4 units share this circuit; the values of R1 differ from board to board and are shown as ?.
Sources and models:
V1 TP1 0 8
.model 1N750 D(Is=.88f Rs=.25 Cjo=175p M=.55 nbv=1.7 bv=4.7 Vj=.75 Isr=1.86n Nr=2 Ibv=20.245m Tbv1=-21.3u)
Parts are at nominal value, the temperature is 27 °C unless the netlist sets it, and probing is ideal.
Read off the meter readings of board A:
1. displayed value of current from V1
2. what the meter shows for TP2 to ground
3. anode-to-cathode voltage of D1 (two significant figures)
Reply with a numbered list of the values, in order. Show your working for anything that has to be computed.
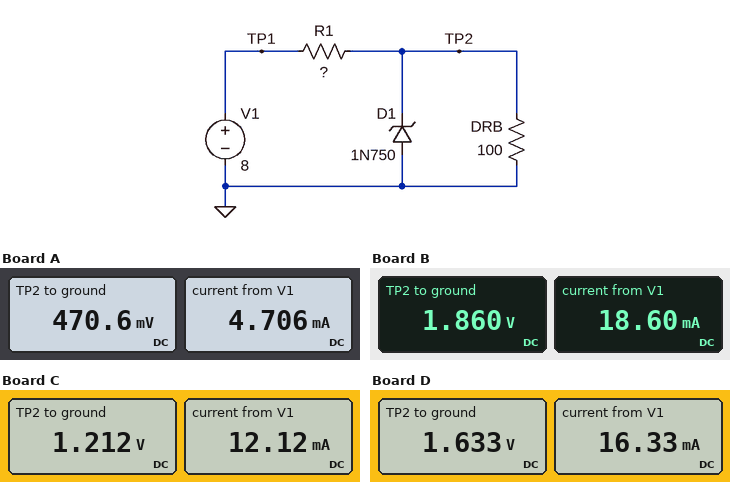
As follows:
1. 4.706 mA
2. 470.6 mV
3. 0 V - 470.6 mV = -470 mV
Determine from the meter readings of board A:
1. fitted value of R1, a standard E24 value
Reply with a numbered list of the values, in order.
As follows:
1. 1.6 kΩ
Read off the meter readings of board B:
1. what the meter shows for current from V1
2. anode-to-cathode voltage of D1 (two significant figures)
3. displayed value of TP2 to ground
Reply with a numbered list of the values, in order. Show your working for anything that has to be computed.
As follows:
1. 18.60 mA
2. 0 V - 1.86 V = -1.9 V
3. 1.860 V
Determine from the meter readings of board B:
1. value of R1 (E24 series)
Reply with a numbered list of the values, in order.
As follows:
1. 330 Ω
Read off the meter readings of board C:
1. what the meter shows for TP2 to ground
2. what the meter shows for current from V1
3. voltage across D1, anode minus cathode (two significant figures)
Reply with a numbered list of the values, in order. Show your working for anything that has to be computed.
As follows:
1. 1.212 V
2. 12.12 mA
3. 0 V - 1.212 V = -1.2 V
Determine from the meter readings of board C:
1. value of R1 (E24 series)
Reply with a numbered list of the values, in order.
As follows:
1. 560 Ω
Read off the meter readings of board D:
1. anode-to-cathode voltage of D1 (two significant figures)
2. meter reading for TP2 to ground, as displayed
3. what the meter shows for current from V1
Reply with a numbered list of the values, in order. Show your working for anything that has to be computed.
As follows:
1. 0 V - 1.633 V = -1.6 V
2. 1.633 V
3. 16.33 mA
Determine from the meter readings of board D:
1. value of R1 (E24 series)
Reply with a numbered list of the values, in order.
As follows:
1. 390 Ω
